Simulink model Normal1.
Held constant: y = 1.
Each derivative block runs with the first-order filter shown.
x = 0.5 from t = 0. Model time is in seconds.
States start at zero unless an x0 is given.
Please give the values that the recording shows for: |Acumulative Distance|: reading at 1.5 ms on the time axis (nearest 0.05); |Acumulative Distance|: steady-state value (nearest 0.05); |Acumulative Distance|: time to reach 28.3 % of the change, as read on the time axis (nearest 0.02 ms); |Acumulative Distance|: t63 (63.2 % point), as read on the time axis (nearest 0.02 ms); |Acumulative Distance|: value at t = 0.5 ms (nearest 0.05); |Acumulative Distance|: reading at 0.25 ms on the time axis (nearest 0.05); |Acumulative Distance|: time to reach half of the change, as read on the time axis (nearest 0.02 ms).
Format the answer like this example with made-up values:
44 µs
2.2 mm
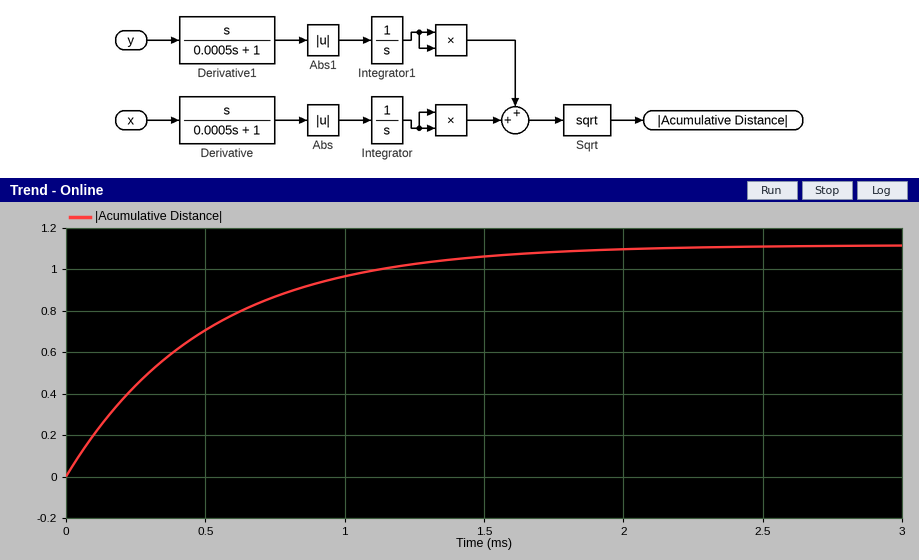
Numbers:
1.05
1.10
0.16 ms
0.50 ms
0.70
0.45
0.34 ms
